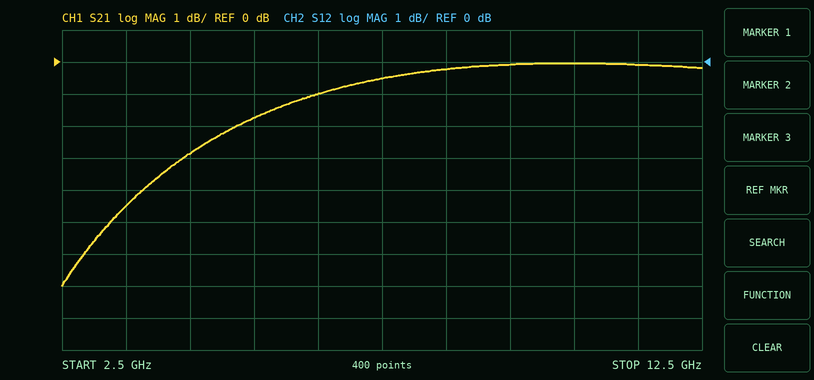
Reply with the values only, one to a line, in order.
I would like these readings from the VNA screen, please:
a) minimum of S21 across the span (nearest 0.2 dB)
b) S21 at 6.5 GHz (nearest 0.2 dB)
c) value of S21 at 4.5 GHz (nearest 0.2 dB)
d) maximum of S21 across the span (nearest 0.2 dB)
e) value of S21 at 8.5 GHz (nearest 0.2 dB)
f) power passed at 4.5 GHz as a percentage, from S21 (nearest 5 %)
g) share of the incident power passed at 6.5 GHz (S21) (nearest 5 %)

-7.0 dB
-1.0 dB
-2.8 dB
0.0 dB
-0.2 dB
50 %
80 %
